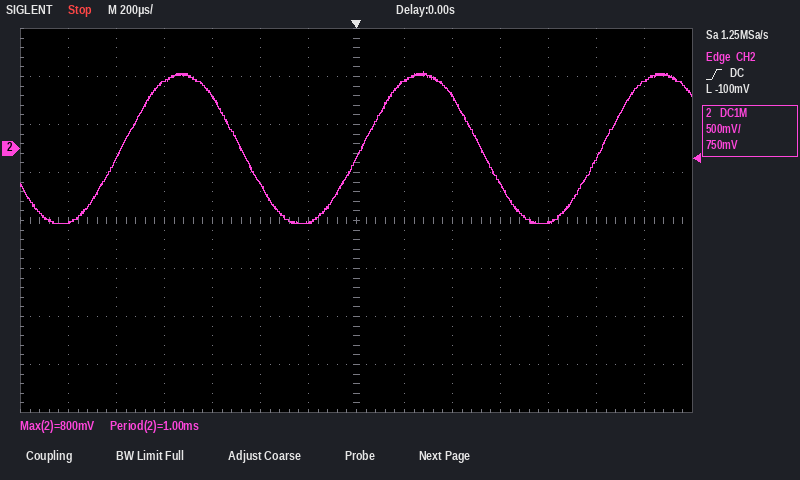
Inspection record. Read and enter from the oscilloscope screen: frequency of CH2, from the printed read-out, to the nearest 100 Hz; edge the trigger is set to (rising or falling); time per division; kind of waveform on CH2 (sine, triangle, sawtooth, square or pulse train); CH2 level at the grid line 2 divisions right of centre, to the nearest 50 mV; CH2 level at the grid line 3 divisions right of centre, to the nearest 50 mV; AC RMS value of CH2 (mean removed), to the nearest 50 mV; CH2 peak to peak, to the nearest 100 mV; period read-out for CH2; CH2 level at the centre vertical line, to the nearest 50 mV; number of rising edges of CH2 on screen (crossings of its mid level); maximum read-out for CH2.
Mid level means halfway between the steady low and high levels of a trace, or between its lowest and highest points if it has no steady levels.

1.0 kHz
rising
200 µs
sine
550 mV
-350 mV
550 mV
1.60 V
1.00 ms
-100 mV
3
800 mV
